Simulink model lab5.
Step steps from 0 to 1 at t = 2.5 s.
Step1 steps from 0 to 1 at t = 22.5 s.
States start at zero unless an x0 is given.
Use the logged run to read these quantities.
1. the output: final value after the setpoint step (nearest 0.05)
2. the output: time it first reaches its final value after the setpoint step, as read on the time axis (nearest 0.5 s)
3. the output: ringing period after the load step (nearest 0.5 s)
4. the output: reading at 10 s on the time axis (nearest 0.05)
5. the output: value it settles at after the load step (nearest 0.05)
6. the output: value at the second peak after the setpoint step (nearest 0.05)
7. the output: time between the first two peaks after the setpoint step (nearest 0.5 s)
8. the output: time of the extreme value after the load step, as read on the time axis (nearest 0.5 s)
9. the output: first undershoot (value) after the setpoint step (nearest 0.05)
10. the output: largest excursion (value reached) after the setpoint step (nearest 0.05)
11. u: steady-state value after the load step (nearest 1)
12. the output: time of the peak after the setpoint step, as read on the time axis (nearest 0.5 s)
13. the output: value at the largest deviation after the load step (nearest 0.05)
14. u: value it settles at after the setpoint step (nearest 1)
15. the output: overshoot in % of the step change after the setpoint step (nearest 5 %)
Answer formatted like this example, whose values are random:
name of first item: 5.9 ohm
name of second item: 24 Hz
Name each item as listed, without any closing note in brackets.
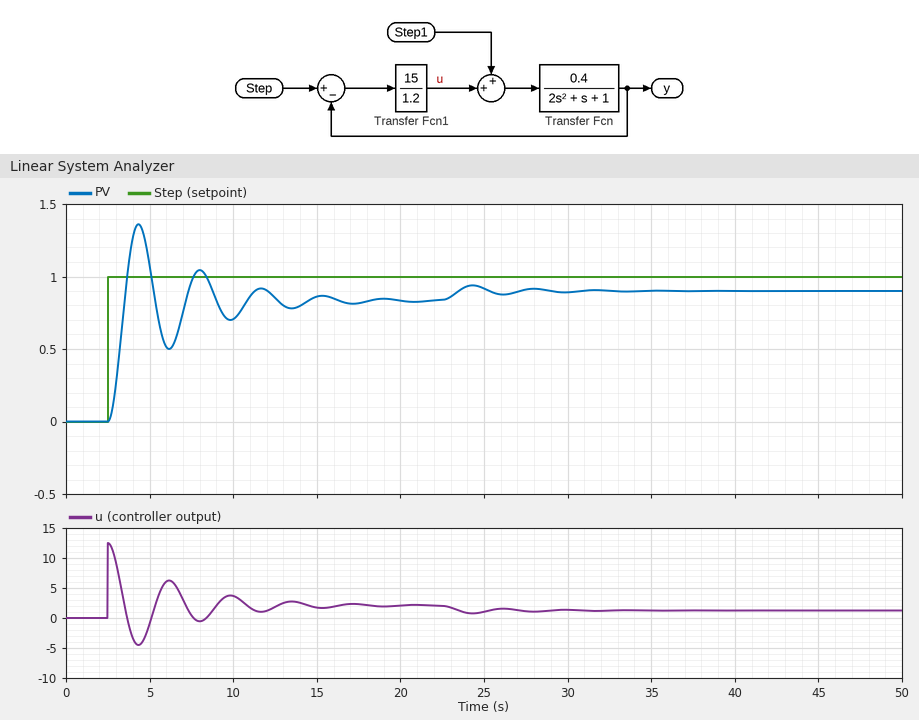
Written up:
the output: final value after the setpoint step: 0.85
the output: time it first reaches its final value after the setpoint step, as read on the time axis: 3.5 s
the output: ringing period after the load step: 3.5 s
the output: reading at 10 s on the time axis: 0.70
the output: value it settles at after the load step: 0.90
the output: value at the second peak after the setpoint step: 1.05
the output: time between the first two peaks after the setpoint step: 3.5 s
the output: time of the extreme value after the load step, as read on the time axis: 24.5 s
the output: first undershoot (value) after the setpoint step: 0.50
the output: largest excursion (value reached) after the setpoint step: 1.35
u: steady-state value after the load step: 1
the output: time of the peak after the setpoint step, as read on the time axis: 4.5 s
the output: value at the largest deviation after the load step: 0.95
u: value it settles at after the setpoint step: 2
the output: overshoot in % of the step change after the setpoint step: 65 %
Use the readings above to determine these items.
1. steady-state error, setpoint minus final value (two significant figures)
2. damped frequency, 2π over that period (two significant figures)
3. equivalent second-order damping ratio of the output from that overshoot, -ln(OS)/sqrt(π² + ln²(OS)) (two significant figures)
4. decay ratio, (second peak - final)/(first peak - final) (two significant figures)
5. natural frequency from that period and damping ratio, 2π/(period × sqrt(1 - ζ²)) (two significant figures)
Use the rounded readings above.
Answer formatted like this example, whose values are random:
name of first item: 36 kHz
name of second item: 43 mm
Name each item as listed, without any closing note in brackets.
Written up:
steady-state error, setpoint minus final value: 0.15
damped frequency, 2π over that period: 1.8 rad/s
equivalent second-order damping ratio of the output from that overshoot, -ln(OS)/sqrt(π² + ln²(OS)): 0.14
decay ratio, (second peak - final)/(first peak - final): 0.40
natural frequency from that period and damping ratio, 2π/(period × sqrt(1 - ζ²)): 1.8 rad/s
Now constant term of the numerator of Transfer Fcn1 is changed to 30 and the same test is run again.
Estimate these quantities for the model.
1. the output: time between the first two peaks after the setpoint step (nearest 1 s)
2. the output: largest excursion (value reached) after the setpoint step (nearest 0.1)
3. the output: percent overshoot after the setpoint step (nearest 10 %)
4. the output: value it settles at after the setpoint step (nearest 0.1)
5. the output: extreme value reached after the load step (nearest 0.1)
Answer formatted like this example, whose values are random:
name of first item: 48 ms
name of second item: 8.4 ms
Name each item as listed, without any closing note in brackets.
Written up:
the output: time between the first two peaks after the setpoint step: 3 s
the output: largest excursion (value reached) after the setpoint step: 1.6
the output: percent overshoot after the setpoint step: 70 %
the output: value it settles at after the setpoint step: 0.9
the output: extreme value reached after the load step: 1.0
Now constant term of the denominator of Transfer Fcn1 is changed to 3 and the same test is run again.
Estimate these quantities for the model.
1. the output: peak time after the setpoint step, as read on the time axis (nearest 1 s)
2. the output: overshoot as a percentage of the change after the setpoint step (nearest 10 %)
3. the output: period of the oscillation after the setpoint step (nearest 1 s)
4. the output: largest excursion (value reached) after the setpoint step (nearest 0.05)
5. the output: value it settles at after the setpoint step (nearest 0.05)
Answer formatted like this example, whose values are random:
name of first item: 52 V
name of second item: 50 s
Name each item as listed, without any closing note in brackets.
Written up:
the output: peak time after the setpoint step, as read on the time axis: 5 s
the output: overshoot as a percentage of the change after the setpoint step: 50 %
the output: period of the oscillation after the setpoint step: 5 s
the output: largest excursion (value reached) after the setpoint step: 1.00
the output: value it settles at after the setpoint step: 0.65
